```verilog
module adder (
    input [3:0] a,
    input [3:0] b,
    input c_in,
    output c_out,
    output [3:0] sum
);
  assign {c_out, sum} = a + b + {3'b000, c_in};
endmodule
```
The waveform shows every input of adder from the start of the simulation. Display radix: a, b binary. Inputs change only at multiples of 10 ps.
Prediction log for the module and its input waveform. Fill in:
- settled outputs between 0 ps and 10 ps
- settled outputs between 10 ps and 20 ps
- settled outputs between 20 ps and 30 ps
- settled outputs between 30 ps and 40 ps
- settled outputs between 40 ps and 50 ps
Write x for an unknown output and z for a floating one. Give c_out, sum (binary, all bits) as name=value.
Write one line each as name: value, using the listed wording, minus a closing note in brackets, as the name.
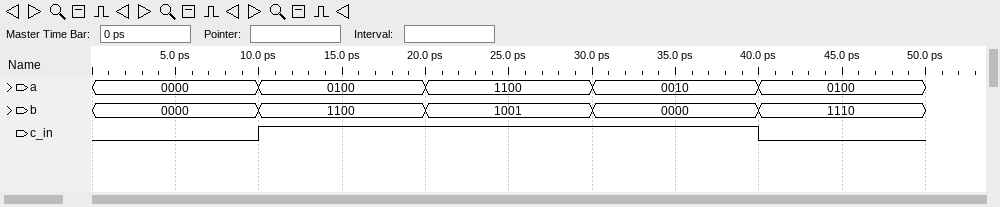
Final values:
settled outputs between 0 ps and 10 ps: c_out=0, sum=0000
settled outputs between 10 ps and 20 ps: c_out=1, sum=0001
settled outputs between 20 ps and 30 ps: c_out=1, sum=0110
settled outputs between 30 ps and 40 ps: c_out=0, sum=0011
settled outputs between 40 ps and 50 ps: c_out=1, sum=0010
